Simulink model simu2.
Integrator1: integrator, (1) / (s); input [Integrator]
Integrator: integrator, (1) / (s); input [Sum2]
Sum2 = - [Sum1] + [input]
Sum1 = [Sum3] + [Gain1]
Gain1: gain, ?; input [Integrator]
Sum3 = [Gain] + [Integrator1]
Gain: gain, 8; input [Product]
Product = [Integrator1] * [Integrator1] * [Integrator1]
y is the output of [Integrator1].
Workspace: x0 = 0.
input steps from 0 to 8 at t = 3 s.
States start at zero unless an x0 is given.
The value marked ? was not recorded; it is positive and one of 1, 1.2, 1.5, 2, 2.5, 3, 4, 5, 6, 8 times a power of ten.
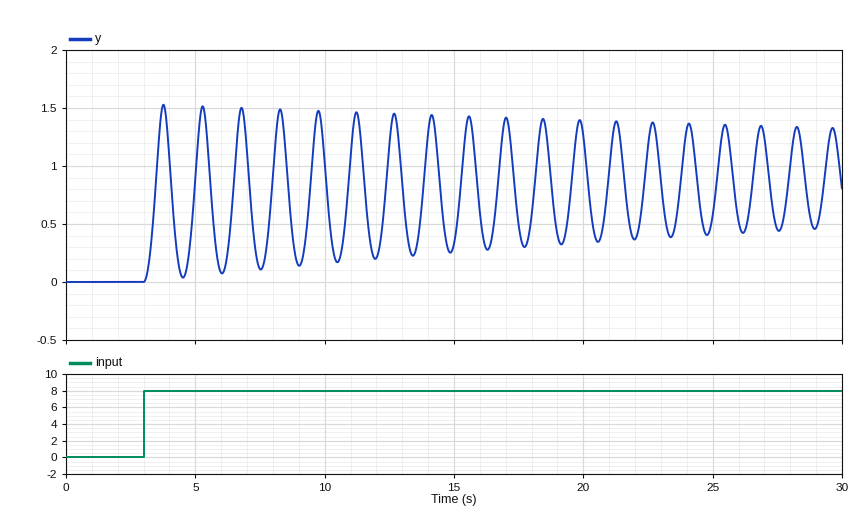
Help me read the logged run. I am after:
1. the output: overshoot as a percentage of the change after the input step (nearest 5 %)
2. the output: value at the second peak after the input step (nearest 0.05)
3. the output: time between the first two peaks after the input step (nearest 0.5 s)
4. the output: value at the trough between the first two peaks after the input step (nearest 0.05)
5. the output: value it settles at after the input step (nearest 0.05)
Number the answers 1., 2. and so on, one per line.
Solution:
1. 60 %
2. 1.50
3. 1.5 s
4. 0.05
5. 0.95
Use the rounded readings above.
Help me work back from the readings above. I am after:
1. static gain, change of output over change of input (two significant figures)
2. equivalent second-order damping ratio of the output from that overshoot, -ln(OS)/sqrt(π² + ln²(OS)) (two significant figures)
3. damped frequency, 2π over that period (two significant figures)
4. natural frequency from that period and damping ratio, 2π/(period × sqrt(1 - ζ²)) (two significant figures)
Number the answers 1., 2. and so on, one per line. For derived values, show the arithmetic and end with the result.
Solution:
1. (0.95 - 0) / (8 - 0) = 0.12
2. ln(0.6) = -0.511; 0.511 / sqrt(9.870 + 0.261) = 0.16
3. 2π / 1.5 = 4.2 rad/s
4. 2π / (1.5 × sqrt(1 - 0.16²)) = 4.2 rad/s
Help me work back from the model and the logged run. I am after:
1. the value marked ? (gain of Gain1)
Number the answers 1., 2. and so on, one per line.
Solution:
1. 0.04
